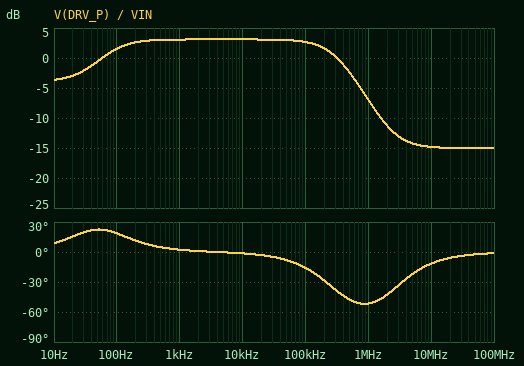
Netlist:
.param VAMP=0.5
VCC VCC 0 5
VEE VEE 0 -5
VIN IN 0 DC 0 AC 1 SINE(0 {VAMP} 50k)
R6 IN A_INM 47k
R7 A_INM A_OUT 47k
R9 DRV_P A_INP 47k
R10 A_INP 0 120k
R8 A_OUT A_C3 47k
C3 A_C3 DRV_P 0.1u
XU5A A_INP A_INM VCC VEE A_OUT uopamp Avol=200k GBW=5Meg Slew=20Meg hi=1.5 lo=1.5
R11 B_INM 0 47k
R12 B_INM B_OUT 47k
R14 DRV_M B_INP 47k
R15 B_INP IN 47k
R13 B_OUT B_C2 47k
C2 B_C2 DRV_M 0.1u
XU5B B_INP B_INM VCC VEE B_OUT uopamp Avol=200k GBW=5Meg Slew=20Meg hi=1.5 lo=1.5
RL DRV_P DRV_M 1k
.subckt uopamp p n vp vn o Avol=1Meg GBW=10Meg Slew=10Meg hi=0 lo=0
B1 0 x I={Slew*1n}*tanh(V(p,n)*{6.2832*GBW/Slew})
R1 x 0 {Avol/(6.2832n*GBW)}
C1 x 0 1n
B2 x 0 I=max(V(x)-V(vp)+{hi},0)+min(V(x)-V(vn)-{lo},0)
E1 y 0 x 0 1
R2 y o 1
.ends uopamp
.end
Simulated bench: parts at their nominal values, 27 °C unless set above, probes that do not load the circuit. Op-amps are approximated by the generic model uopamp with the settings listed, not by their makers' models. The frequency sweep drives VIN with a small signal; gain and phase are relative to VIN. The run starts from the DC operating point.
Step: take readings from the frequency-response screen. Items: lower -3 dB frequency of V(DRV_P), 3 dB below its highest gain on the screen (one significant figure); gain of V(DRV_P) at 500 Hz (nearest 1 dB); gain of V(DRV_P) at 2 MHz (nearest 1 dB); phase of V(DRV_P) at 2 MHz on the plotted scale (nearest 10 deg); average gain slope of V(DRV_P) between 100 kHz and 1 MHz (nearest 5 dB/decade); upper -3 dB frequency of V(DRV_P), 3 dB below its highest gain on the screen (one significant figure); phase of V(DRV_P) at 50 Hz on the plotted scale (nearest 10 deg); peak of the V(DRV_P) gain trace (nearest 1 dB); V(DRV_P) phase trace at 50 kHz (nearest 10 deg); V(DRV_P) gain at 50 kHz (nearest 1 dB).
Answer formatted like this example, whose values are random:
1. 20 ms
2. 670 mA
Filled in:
1. 60 Hz
2. 3 dB
3. -11 dB
4. -40 deg
5. -10 dB/decade
6. 300 kHz
7. 20 deg
8. 3 dB
9. -10 deg
10. 3 dB
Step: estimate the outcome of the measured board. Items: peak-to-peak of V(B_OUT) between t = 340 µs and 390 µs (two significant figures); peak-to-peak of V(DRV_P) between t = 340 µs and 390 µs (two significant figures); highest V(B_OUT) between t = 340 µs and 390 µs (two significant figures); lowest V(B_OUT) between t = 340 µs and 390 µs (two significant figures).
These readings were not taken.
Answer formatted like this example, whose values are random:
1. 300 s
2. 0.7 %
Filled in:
1. 2.4 V
2. 1.4 V
3. 1.2 V
4. -1.2 V
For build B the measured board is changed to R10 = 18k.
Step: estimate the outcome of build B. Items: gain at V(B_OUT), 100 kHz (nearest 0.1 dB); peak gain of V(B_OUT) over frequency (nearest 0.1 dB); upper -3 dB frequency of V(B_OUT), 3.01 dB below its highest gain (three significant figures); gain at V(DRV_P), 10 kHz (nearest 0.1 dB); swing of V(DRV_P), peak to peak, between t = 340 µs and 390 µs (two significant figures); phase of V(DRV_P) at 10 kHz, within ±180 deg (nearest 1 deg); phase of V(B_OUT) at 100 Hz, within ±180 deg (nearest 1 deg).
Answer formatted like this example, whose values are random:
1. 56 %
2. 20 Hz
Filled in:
1. 2.4 dB
2. 3.0 dB
3. 1.75 MHz
4. -10.7 dB
5. 290 mV
6. 0 deg
7. -1 deg
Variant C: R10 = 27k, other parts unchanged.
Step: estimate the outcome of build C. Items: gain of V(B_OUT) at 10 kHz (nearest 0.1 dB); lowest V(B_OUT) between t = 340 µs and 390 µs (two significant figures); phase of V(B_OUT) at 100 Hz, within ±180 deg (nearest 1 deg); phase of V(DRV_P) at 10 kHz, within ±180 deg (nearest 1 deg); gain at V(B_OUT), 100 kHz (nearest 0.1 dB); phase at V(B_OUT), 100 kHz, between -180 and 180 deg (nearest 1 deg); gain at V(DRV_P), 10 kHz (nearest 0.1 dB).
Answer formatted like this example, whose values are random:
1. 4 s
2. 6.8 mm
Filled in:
1. 2.8 dB
2. -690 mV
3. -1 deg
4. 0 deg
5. 2.7 dB
6. -3 deg
7. -9.2 dB
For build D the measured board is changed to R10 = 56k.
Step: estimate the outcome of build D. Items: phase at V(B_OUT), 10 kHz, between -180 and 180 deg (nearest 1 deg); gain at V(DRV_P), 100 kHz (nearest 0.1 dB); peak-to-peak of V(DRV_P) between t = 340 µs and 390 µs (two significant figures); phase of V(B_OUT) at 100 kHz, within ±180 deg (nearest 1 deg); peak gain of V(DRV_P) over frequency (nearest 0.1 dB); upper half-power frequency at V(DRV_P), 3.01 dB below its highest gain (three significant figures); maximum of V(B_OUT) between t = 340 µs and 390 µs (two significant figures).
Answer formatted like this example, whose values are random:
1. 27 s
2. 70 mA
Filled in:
1. 0 deg
2. -5.1 dB
3. 560 mV
4. -4 deg
5. -5.0 dB
6. 797 kHz
7. 790 mV
